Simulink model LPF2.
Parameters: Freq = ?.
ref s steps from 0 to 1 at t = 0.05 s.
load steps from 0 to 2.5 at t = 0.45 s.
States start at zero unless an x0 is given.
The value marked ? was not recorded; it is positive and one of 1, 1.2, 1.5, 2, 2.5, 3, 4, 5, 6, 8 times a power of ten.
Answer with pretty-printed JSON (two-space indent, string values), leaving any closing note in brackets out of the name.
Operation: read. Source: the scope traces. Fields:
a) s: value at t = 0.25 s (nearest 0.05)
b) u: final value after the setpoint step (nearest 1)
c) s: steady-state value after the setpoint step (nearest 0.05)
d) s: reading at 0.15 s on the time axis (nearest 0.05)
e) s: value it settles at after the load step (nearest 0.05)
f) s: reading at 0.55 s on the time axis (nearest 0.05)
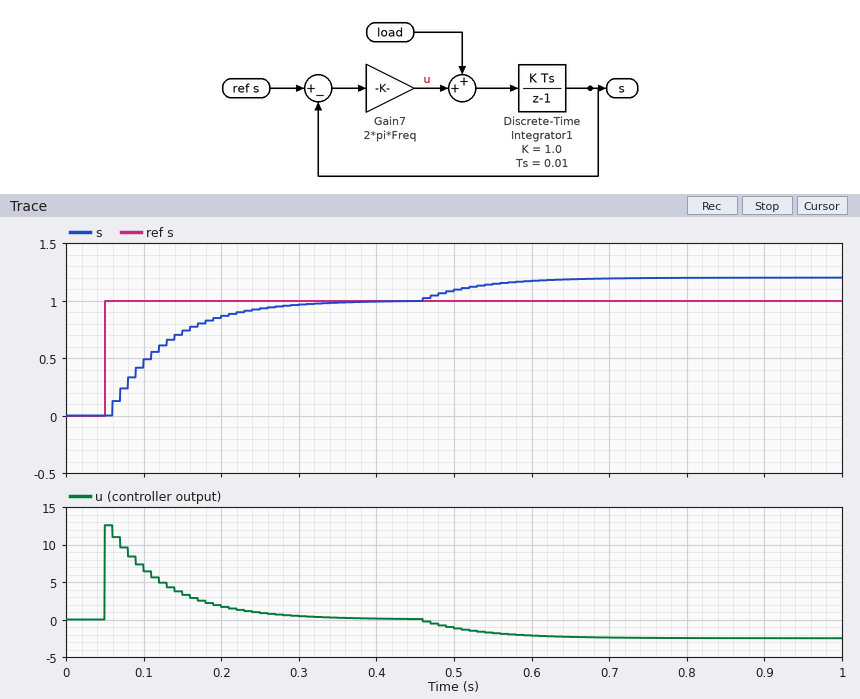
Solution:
{
  "s: value at t = 0.25 s": "0.95",
  "u: final value after the setpoint step": "0",
  "s: steady-state value after the setpoint step": "1.00",
  "s: reading at 0.15 s on the time axis": "0.75",
  "s: value it settles at after the load step": "1.20",
  "s: reading at 0.55 s on the time axis": "1.15"
}
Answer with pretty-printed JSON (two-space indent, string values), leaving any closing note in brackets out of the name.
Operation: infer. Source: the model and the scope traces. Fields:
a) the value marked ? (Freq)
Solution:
{
  "the value marked ?": "2"
}
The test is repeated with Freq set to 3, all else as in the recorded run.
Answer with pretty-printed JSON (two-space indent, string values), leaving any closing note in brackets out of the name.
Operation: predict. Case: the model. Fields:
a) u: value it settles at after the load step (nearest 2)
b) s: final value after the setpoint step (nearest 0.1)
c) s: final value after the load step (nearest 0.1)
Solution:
{
  "u: value it settles at after the load step": "-2",
  "s: final value after the setpoint step": "1.0",
  "s: final value after the load step": "1.1"
}
